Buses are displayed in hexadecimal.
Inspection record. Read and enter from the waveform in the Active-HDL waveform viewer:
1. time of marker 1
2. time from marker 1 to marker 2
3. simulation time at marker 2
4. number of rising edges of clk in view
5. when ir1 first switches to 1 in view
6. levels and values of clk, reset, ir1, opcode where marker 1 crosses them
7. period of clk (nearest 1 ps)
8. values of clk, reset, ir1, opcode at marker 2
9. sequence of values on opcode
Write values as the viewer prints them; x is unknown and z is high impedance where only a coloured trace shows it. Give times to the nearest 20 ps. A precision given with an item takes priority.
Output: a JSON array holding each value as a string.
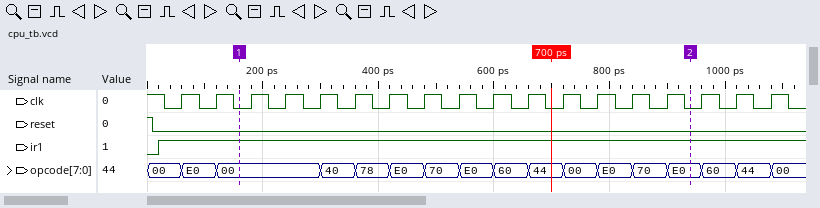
["160 ps", "780 ps", "940 ps", "18", "20 ps", "clk=0, reset=0, ir1=1, opcode=00", "60 ps", "clk=0, reset=0, ir1=1, opcode=E0", "00, E0, 00, 40, 78, E0, 70, E0, 60, 44, 00, E0, 70, E0, 60, 44, 00"]
